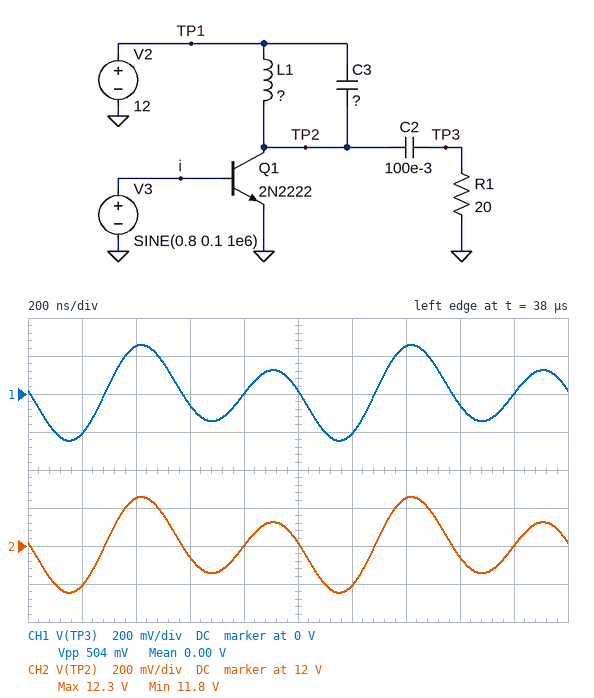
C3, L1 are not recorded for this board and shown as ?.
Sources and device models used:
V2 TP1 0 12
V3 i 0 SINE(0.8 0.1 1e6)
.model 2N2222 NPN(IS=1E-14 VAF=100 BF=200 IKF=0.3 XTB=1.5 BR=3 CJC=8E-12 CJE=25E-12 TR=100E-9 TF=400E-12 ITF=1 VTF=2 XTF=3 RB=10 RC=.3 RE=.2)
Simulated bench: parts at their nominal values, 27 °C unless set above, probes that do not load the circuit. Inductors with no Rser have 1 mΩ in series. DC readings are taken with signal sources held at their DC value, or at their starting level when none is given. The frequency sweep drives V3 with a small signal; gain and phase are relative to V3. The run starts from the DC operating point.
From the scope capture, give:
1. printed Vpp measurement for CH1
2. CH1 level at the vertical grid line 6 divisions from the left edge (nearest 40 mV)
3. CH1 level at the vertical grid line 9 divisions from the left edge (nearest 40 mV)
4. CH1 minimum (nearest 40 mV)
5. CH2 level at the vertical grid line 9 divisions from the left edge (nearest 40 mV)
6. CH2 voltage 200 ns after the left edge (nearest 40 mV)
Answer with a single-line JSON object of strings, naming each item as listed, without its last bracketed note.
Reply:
{"printed Vpp measurement for CH1": "504 mV", "CH1 level at the vertical grid line 6 divisions from the left edge": "-200 mV", "CH1 level at the vertical grid line 9 divisions from the left edge": "0 V", "CH1 minimum": "-240 mV", "CH2 level at the vertical grid line 9 divisions from the left edge": "12.00 V", "CH2 voltage 200 ns after the left edge": "11.80 V"}
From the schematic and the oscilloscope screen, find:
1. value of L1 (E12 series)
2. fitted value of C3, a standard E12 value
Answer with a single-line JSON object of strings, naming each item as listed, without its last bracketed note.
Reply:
{"value of L1": "68 nH", "fitted value of C3, a standard E12 value": "82 nF"}
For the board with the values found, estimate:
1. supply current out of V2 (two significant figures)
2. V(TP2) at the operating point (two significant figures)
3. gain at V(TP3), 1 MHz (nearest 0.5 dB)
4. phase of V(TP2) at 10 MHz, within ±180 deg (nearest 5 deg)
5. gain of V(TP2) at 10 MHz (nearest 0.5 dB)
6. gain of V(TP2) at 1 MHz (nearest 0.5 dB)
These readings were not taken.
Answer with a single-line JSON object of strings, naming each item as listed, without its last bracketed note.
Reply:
{"supply current out of V2": "93 mA", "V(TP2) at the operating point": "12 V", "gain at V(TP3), 1 MHz": "-1.0 dB", "phase of V(TP2) at 10 MHz, within ±180 deg": "65 deg", "gain of V(TP2) at 10 MHz": "-10.5 dB", "gain of V(TP2) at 1 MHz": "-1.0 dB"}
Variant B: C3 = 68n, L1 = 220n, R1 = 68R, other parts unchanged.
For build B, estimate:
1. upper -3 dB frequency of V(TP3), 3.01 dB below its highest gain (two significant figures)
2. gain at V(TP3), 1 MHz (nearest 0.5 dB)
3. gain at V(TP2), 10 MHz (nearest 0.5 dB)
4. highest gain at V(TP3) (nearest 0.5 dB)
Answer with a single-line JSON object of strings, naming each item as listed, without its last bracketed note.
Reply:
{"upper -3 dB frequency of V(TP3), 3.01 dB below its highest gain": "1.3 MHz", "gain at V(TP3), 1 MHz": "15.0 dB", "gain at V(TP2), 10 MHz": "-9.0 dB", "highest gain at V(TP3)": "40.5 dB"}
